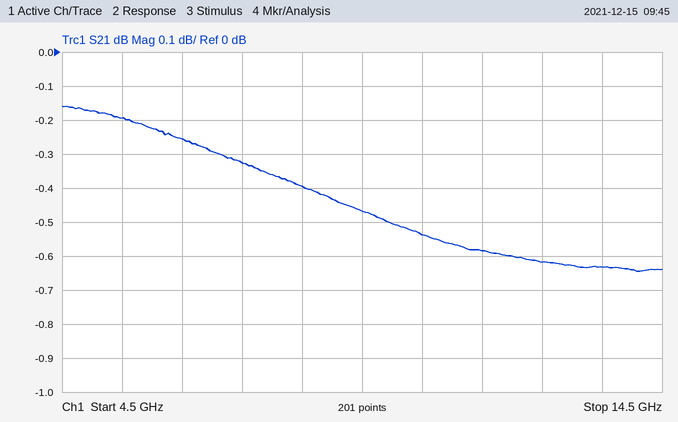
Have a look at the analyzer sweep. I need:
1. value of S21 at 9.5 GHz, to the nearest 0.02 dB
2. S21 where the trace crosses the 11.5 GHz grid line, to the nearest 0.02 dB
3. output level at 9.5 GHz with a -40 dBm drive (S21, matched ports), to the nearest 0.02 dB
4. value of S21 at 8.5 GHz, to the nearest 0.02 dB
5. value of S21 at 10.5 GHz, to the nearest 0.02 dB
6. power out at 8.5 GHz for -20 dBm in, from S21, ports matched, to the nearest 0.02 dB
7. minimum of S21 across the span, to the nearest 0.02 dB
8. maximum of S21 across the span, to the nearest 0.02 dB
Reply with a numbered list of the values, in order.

1. -0.46 dB
2. -0.58 dB
3. -40.46 dBm
4. -0.40 dB
5. -0.54 dB
6. -20.40 dBm
7. -0.64 dB
8. -0.16 dB
